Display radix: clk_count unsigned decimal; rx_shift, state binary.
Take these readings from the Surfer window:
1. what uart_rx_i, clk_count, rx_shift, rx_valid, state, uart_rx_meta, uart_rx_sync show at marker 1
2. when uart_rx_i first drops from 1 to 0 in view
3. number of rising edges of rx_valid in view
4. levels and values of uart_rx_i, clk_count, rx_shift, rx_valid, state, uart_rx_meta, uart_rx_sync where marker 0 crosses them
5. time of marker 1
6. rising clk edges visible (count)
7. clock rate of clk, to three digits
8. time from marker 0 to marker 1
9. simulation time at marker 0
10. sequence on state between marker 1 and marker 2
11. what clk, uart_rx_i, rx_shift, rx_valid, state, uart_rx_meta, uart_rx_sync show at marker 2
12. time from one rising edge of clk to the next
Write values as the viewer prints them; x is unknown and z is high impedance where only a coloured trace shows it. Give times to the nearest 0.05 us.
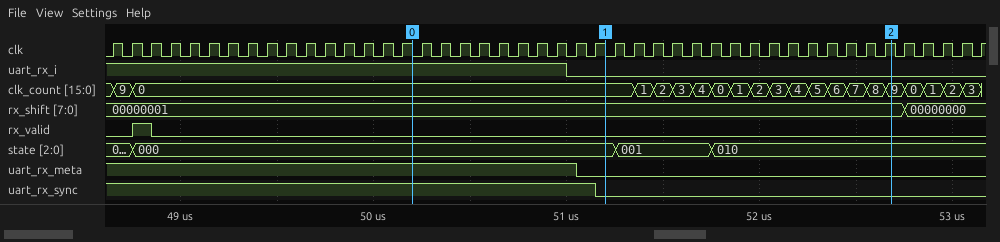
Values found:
uart_rx_i=0, clk_count=0, rx_shift=00000001, rx_valid=0, state=000, uart_rx_meta=0, uart_rx_sync=0
51 us
1
uart_rx_i=1, clk_count=0, rx_shift=00000001, rx_valid=0, state=000, uart_rx_meta=1, uart_rx_sync=1
51.2 us
46
10.0 MHz
1 us
50.2 us
000, 001, 010
clk=1, uart_rx_i=0, rx_shift=00000001, rx_valid=0, state=010, uart_rx_meta=0, uart_rx_sync=0
0.1 us
